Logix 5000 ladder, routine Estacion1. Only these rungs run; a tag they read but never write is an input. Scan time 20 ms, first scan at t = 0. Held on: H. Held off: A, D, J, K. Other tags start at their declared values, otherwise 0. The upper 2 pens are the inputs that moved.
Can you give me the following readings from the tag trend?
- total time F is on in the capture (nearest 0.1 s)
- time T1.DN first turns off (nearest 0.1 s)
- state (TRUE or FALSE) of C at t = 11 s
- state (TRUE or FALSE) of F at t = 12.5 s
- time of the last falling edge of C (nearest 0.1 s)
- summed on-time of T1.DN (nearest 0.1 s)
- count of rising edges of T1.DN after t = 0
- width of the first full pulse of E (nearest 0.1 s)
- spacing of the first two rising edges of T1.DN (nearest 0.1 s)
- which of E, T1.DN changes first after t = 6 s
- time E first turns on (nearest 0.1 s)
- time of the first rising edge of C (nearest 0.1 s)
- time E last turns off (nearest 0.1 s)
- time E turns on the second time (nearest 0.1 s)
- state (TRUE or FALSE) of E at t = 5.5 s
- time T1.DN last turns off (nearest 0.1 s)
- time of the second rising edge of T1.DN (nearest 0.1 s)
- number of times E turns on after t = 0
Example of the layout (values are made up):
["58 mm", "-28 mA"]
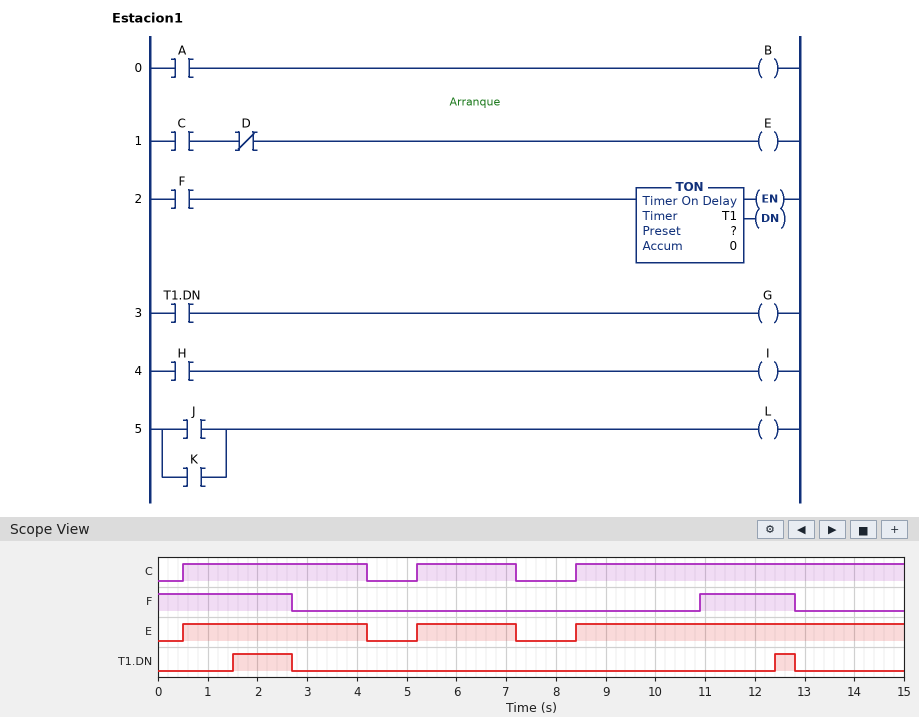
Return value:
["4.6 s", "2.7 s", "TRUE", "TRUE", "7.2 s", "1.6 s", "2", "3.7 s", "10.9 s", "E", "0.5 s", "0.5 s", "7.2 s", "5.2 s", "TRUE", "12.8 s", "12.4 s", "3"]
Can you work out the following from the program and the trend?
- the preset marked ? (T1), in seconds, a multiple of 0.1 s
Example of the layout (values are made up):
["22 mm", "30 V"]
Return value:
["1.5 s"]
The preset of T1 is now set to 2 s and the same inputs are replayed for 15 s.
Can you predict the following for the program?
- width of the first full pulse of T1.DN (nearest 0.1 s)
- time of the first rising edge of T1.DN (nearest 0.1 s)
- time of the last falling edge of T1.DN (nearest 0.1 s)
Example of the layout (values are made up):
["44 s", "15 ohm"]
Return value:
["0.7 s", "2.0 s", "2.7 s"]
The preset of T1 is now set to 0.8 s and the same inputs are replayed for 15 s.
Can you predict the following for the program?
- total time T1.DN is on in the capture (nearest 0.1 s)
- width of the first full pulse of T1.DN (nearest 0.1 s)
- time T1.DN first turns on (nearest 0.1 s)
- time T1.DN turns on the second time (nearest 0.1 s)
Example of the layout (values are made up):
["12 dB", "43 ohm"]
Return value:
["3.0 s", "1.9 s", "0.8 s", "11.7 s"]
